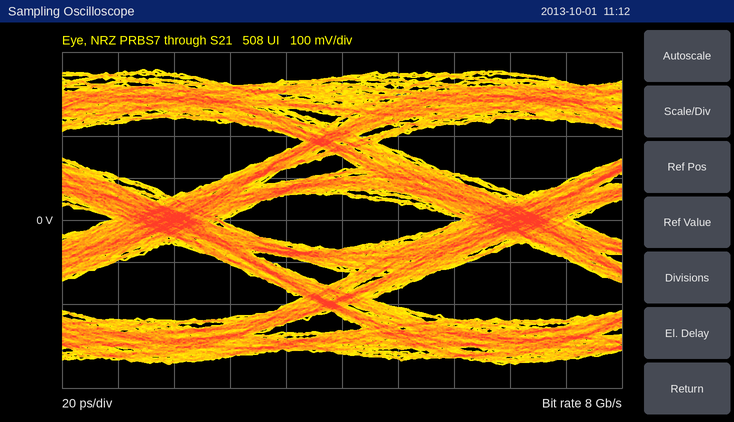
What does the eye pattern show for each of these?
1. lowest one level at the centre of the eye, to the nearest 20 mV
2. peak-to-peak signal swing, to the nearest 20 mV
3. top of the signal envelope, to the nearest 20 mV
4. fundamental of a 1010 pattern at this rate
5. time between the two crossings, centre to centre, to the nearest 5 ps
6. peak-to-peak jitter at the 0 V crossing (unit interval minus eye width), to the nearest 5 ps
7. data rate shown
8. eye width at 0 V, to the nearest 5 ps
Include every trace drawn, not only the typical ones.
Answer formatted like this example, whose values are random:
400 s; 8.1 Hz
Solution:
60 mV; 700 mV; 360 mV; 4 GHz; 125 ps; 40 ps; 8 Gb/s; 85 ps
